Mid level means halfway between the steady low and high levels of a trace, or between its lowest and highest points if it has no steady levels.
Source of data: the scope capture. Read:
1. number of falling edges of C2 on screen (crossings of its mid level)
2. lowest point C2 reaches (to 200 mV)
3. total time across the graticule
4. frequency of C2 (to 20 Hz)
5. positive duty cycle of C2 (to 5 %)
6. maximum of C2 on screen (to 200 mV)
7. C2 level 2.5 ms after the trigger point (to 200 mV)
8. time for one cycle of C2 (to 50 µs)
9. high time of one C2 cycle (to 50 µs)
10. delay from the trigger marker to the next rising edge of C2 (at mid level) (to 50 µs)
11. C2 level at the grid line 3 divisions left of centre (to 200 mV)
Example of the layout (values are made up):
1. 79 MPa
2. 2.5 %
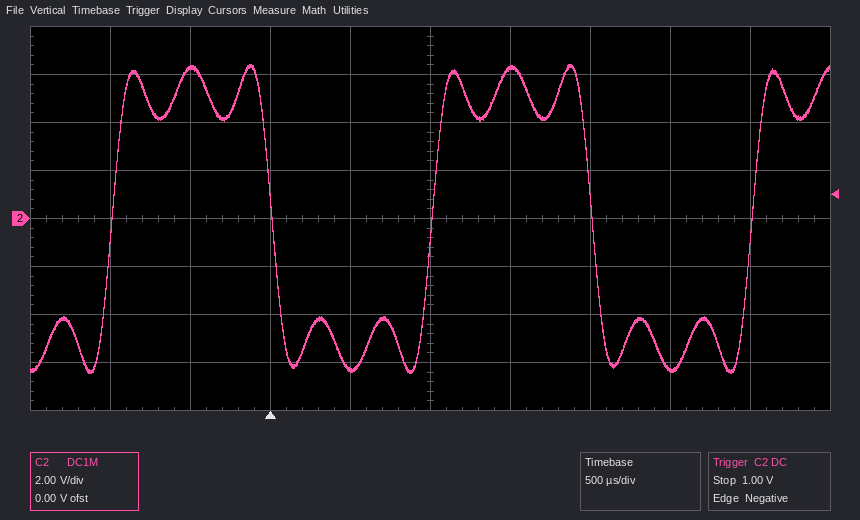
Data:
1. 2
2. -6.4 V
3. 5 ms
4. 500 Hz
5. 50 %
6. 6.4 V
7. -6.2 V
8. 2.00 ms
9. 1.00 ms
10. 1.00 ms
11. 6.2 V
